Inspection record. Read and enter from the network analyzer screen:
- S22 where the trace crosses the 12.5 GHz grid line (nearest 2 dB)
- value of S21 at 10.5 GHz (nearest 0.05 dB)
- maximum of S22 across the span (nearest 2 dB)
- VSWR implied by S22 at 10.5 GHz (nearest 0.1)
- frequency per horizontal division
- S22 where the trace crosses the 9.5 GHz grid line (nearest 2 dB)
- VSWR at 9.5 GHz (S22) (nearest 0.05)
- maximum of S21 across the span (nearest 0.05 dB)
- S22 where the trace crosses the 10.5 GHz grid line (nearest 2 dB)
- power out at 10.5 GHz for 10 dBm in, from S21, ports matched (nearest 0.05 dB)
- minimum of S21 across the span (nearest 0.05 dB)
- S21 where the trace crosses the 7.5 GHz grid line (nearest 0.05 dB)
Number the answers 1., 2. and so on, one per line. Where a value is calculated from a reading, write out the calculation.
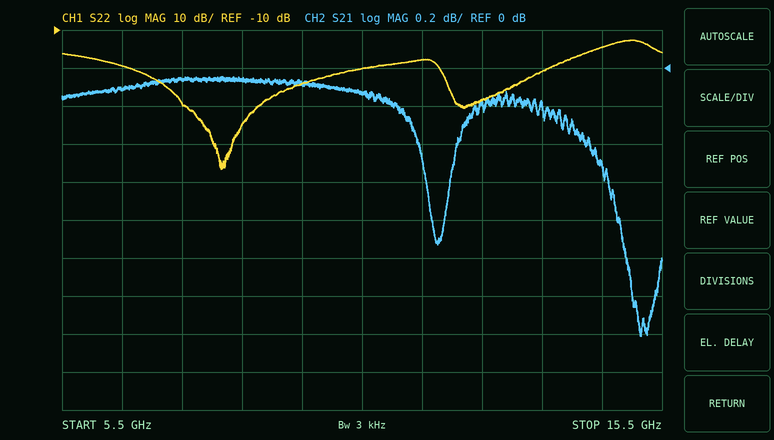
1. -28 dB
2. -0.15 dB
3. -12 dB
4. |Γ| = 10^(-20/20) = 0.1000; VSWR = (1 + 0.1000)/(1 − 0.1000) ≈ 1.2
5. 1 GHz
6. -24 dB
7. |Γ| = 10^(-24/20) = 0.0631; VSWR = (1 + 0.0631)/(1 − 0.0631) ≈ 1.13, so 1.15 to the nearest 0.05
8. -0.05 dB
9. -20 dB
10. 10 dBm + (-0.15 dB) = 9.85 dBm
11. -1.40 dB
12. -0.05 dB
